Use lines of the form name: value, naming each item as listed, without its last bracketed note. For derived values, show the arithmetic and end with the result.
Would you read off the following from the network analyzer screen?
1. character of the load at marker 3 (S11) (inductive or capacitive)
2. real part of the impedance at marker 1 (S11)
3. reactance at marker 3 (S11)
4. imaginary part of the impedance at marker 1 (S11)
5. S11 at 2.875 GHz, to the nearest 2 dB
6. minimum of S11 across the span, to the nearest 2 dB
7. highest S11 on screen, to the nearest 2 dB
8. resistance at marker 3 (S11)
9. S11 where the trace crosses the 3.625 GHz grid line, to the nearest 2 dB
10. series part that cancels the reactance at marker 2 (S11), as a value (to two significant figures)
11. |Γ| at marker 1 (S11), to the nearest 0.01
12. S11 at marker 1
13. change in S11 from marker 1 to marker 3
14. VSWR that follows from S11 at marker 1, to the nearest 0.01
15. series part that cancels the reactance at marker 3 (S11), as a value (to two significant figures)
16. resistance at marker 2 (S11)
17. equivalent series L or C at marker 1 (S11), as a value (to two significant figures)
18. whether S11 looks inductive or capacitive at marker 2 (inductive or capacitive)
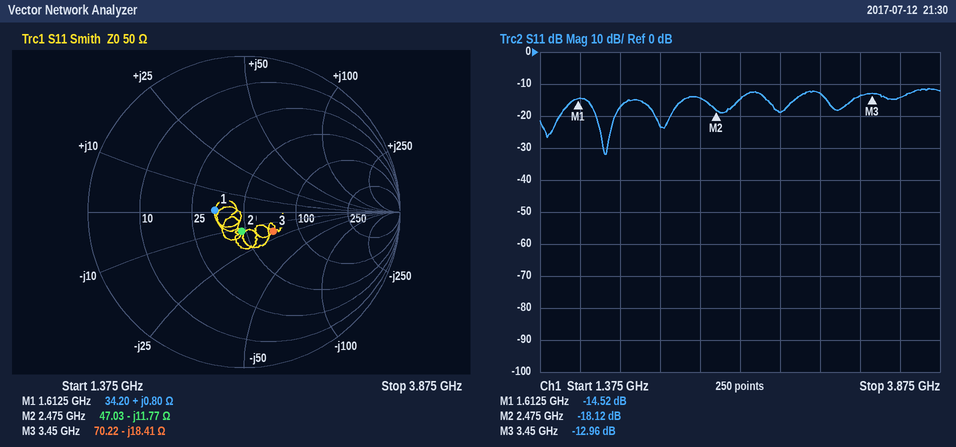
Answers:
character of the load at marker 3 (S11): capacitive
real part of the impedance at marker 1: 34.20 Ω
reactance at marker 3: -18.41 Ω
imaginary part of the impedance at marker 1: +0.80 Ω
S11 at 2.875 GHz, to the nearest 2 dB: -18 dB
minimum of S11 across the span, to the nearest 2 dB: -32 dB
highest S11 on screen, to the nearest 2 dB: -12 dB
resistance at marker 3: 70.22 Ω
S11 where the trace crosses the 3.625 GHz grid line, to the nearest 2 dB: -14 dB
series part that cancels the reactance at marker 2 (S11), as a value: L = 11.77 Ω/(2π × 2.475 GHz) ≈ 757 pH, so 760 pH to two significant figures
|Γ| at marker 1 (S11), to the nearest 0.01: 0.19
S11 at marker 1: -14.52 dB
change in S11 from marker 1 to marker 3: -12.96 − (-14.52) = 1.56 dB
VSWR that follows from S11 at marker 1, to the nearest 0.01: (1 + 0.1879)/(1 − 0.1879) ≈ 1.46
series part that cancels the reactance at marker 3 (S11), as a value: L = 18.41 Ω/(2π × 3.45 GHz) ≈ 849 pH, so 850 pH to two significant figures
resistance at marker 2: 47.03 Ω
equivalent series L or C at marker 1 (S11), as a value: L = 0.8 Ω/(2π × 1.6125 GHz) ≈ 79 pH
whether S11 looks inductive or capacitive at marker 2: capacitive
